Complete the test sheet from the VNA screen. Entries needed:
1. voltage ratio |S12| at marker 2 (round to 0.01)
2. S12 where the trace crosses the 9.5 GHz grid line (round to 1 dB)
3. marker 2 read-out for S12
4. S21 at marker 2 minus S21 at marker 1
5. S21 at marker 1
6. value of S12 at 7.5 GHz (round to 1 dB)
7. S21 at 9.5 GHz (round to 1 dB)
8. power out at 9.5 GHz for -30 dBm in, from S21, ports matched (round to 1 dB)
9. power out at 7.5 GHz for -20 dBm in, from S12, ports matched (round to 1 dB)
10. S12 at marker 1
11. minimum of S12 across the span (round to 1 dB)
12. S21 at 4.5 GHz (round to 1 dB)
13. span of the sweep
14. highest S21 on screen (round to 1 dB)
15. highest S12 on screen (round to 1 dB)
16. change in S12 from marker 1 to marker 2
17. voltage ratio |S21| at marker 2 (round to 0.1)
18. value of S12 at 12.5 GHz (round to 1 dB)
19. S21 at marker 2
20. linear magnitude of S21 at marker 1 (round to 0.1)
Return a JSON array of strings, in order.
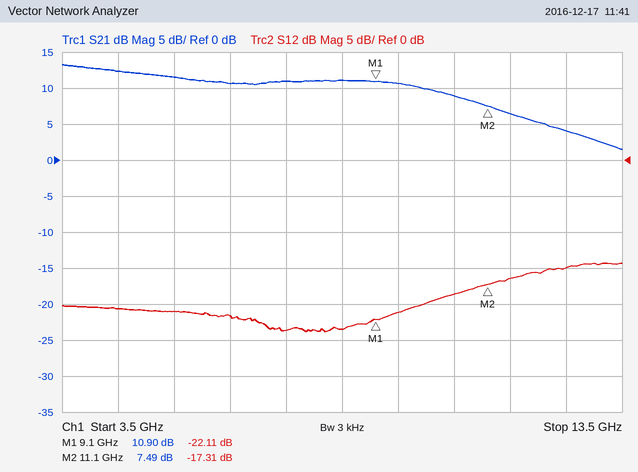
["0.14", "-21 dB", "-17.31 dB", "-3.41 dB", "10.90 dB", "-24 dB", "11 dB", "-19 dBm", "-44 dBm", "-22.11 dB", "-24 dB", "12 dB", "10 GHz", "13 dB", "-14 dB", "4.80 dB", "2.4", "-15 dB", "7.49 dB", "3.5"]
